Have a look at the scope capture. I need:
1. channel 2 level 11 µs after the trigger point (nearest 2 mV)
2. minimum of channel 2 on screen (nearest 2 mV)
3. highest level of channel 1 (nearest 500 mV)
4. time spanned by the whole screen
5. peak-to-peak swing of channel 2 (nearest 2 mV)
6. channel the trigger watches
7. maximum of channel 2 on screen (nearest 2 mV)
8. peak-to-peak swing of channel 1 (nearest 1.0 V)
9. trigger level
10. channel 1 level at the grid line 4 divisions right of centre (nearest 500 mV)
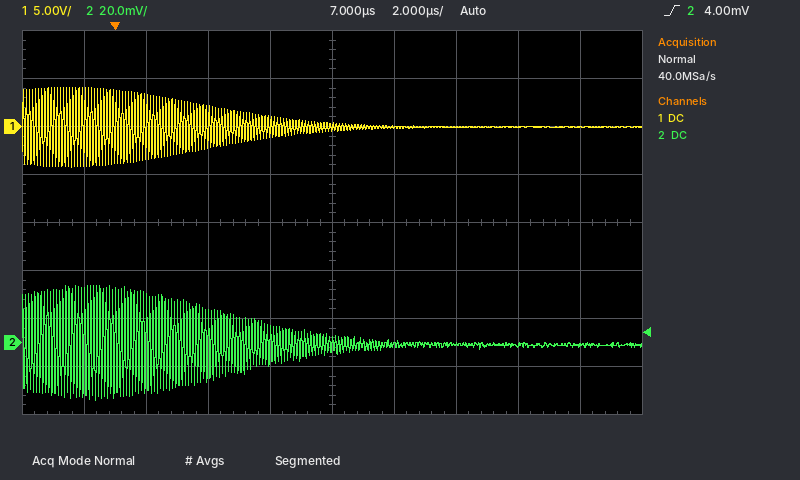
0 mV
-24 mV
4.0 V
20 µs
48 mV
channel 2
24 mV
8.0 V
4.00 mV
0.0 V
